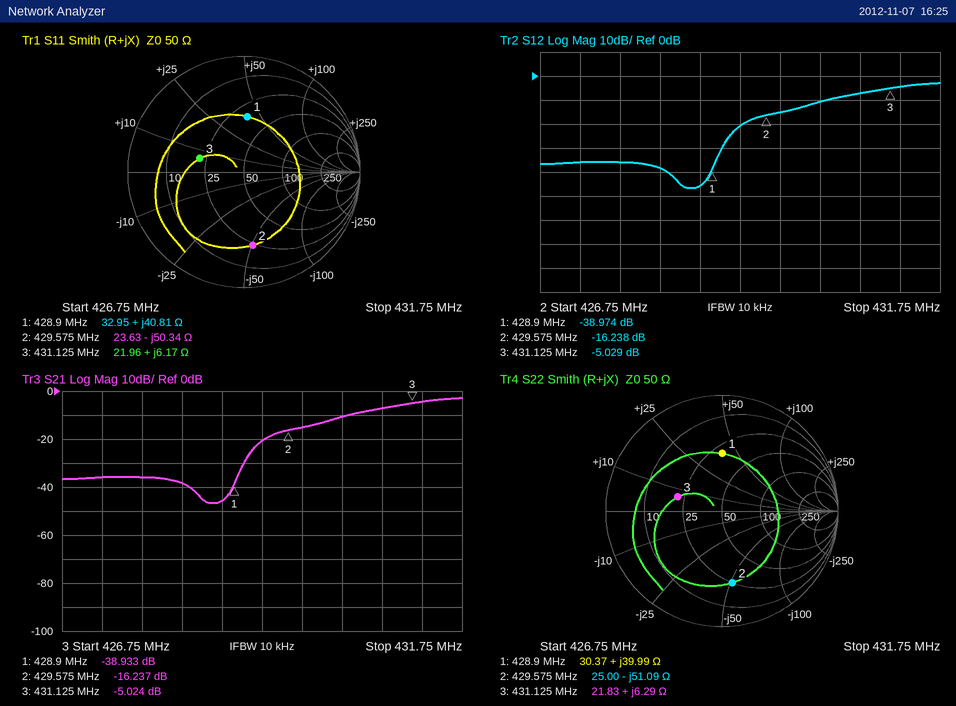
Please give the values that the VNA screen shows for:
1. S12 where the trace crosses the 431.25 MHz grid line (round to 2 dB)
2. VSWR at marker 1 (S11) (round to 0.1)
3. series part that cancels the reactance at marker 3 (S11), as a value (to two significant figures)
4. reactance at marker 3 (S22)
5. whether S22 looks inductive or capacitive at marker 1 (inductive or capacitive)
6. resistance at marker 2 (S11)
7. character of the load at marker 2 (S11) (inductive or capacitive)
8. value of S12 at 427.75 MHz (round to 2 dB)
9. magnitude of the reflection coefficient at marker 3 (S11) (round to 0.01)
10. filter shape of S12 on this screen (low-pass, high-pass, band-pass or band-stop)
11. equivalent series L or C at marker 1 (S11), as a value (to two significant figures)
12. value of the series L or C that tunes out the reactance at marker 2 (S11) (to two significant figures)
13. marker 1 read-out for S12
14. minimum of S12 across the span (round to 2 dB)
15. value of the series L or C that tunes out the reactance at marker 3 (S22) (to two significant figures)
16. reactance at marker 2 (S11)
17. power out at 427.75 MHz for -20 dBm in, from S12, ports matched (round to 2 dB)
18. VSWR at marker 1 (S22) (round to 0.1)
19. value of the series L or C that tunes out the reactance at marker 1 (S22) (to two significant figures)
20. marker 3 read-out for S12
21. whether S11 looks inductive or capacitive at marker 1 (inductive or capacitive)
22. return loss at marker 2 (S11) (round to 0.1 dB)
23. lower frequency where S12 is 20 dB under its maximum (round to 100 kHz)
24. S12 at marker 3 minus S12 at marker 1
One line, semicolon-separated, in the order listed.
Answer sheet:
-4 dB; 2.8; 60 pF; +6.29 Ω; inductive; 23.63 Ω; capacitive; -36 dB; 0.40; high-pass; 15 nH; 19 nH; -38.974 dB; -46 dB; 59 pF; -50.34 Ω; -56 dBm; 3.0; 9.3 pF; -5.029 dB; inductive; 3.9 dB; 429.2 MHz; 33.945 dB
